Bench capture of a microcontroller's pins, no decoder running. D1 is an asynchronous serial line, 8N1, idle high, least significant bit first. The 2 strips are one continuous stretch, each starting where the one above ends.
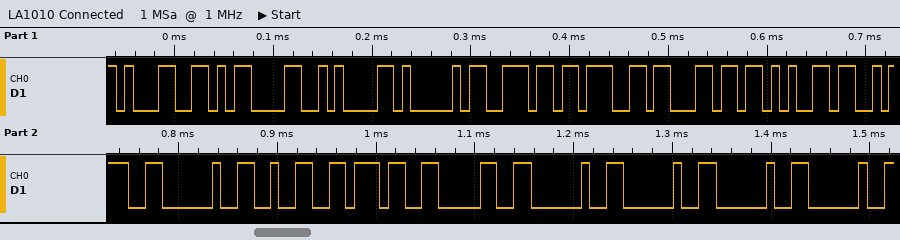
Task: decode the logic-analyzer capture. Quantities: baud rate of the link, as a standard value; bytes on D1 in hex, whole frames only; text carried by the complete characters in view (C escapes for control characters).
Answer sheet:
115200 baud
31 0D 0A 41 6E 67 6C 65 3A 20 32 37 30 20 20 20 20
"1\r\nAngle: 270    "
